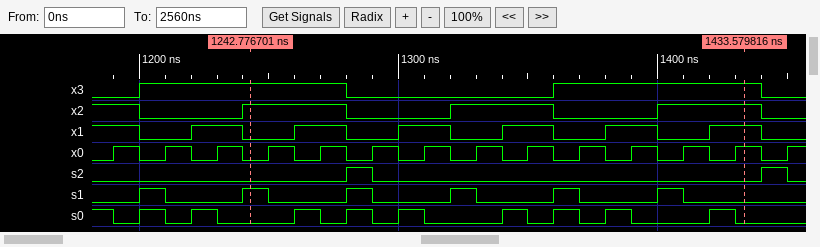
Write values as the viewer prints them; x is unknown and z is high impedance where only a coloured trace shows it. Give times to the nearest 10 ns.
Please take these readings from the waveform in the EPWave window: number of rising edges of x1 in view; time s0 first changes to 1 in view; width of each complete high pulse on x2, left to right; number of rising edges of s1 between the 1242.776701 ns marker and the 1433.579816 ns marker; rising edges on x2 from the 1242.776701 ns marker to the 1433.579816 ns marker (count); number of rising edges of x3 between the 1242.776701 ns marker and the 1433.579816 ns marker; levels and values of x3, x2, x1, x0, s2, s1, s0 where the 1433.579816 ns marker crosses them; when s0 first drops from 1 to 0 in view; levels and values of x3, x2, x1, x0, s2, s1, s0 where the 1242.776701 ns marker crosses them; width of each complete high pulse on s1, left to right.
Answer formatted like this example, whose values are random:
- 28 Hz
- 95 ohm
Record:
- 6
- 1200 ns
- 40 ns, 40 ns, 40 ns
- 4
- 2
- 1
- x3=1, x2=1, x1=1, x0=1, s2=0, s1=0, s0=0
- 1190 ns
- x3=1, x2=1, x1=0, x0=0, s2=0, s1=1, s0=0
- 10 ns, 10 ns, 10 ns, 10 ns, 10 ns, 10 ns
